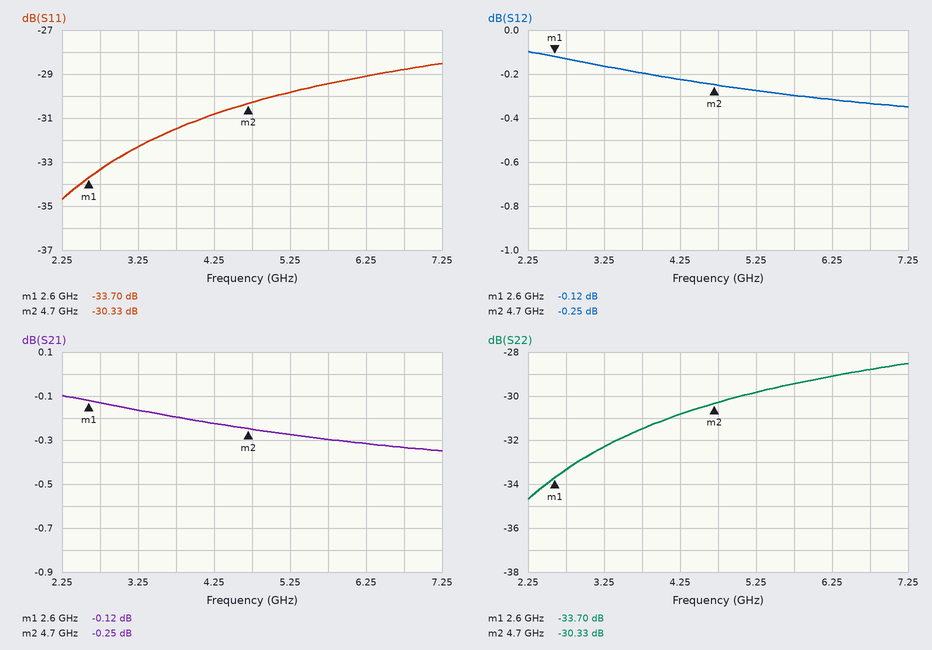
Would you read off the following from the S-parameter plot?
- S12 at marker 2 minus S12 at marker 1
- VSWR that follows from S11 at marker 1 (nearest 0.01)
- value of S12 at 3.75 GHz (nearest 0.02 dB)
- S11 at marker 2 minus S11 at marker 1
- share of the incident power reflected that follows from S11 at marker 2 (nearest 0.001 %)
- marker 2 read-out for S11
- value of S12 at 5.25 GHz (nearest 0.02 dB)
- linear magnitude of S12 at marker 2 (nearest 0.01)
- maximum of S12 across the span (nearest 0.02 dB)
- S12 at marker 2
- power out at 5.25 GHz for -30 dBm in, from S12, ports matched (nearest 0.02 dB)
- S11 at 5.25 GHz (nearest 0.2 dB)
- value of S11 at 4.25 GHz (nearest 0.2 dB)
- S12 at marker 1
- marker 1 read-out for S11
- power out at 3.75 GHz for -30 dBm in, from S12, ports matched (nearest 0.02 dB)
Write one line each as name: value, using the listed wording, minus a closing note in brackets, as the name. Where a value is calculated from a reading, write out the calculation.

S12 at marker 2 minus S12 at marker 1: -0.25 − (-0.12) = -0.13 dB
VSWR that follows from S11 at marker 1: (1 + 0.0207)/(1 − 0.0207) ≈ 1.04
value of S12 at 3.75 GHz: -0.20 dB
S11 at marker 2 minus S11 at marker 1: -30.33 − (-33.7) = 3.37 dB
share of the incident power reflected that follows from S11 at marker 2: 10^(-30.33/10) ≈ 0.093 %
marker 2 read-out for S11: -30.33 dB
value of S12 at 5.25 GHz: -0.28 dB
linear magnitude of S12 at marker 2: 10^(-0.25/20) ≈ 0.97
maximum of S12 across the span: -0.10 dB
S12 at marker 2: -0.25 dB
power out at 5.25 GHz for -30 dBm in, from S12, ports matched: -30 dBm + (-0.28 dB) = -30.28 dBm
S11 at 5.25 GHz: -29.8 dB
value of S11 at 4.25 GHz: -30.8 dB
S12 at marker 1: -0.12 dB
marker 1 read-out for S11: -33.70 dB
power out at 3.75 GHz for -30 dBm in, from S12, ports matched: -30 dBm + (-0.20 dB) = -30.20 dBm
